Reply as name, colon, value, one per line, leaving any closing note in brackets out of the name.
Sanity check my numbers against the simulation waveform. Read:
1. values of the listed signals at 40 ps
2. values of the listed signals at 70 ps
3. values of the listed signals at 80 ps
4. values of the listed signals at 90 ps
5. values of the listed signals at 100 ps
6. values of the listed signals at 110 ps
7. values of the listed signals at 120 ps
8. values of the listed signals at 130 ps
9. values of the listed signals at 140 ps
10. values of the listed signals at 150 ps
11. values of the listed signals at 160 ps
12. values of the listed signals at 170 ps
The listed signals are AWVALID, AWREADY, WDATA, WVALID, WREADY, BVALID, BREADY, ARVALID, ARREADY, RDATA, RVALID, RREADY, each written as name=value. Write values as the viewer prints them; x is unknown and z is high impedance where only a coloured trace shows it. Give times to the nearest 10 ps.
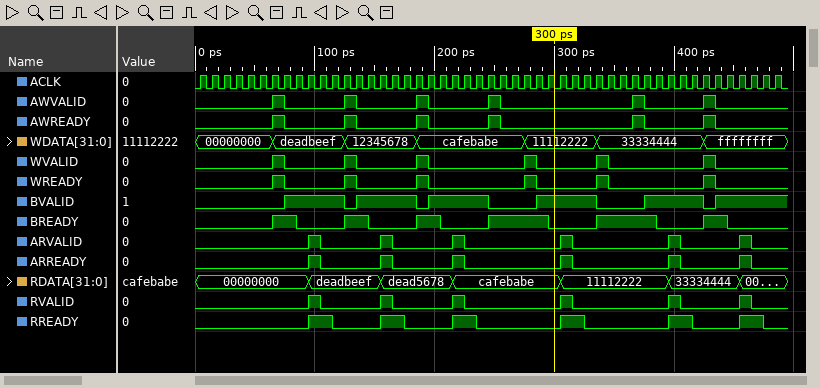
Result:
values of the listed signals at 40 ps: AWVALID=0, AWREADY=0, WDATA=00000000, WVALID=0, WREADY=0, BVALID=0, BREADY=0, ARVALID=0, ARREADY=0, RDATA=00000000, RVALID=0, RREADY=0
values of the listed signals at 70 ps: AWVALID=1, AWREADY=1, WDATA=deadbeef, WVALID=1, WREADY=1, BVALID=0, BREADY=1, ARVALID=0, ARREADY=0, RDATA=00000000, RVALID=0, RREADY=0
values of the listed signals at 80 ps: AWVALID=0, AWREADY=0, WDATA=deadbeef, WVALID=0, WREADY=0, BVALID=1, BREADY=1, ARVALID=0, ARREADY=0, RDATA=00000000, RVALID=0, RREADY=0
values of the listed signals at 90 ps: AWVALID=0, AWREADY=0, WDATA=deadbeef, WVALID=0, WREADY=0, BVALID=1, BREADY=0, ARVALID=0, ARREADY=0, RDATA=00000000, RVALID=0, RREADY=0
values of the listed signals at 100 ps: AWVALID=0, AWREADY=0, WDATA=deadbeef, WVALID=0, WREADY=0, BVALID=1, BREADY=0, ARVALID=1, ARREADY=1, RDATA=deadbeef, RVALID=1, RREADY=1
values of the listed signals at 110 ps: AWVALID=0, AWREADY=0, WDATA=deadbeef, WVALID=0, WREADY=0, BVALID=1, BREADY=0, ARVALID=0, ARREADY=0, RDATA=deadbeef, RVALID=0, RREADY=1
values of the listed signals at 120 ps: AWVALID=0, AWREADY=0, WDATA=deadbeef, WVALID=0, WREADY=0, BVALID=1, BREADY=0, ARVALID=0, ARREADY=0, RDATA=deadbeef, RVALID=0, RREADY=0
values of the listed signals at 130 ps: AWVALID=1, AWREADY=1, WDATA=12345678, WVALID=1, WREADY=1, BVALID=0, BREADY=1, ARVALID=0, ARREADY=0, RDATA=deadbeef, RVALID=0, RREADY=0
values of the listed signals at 140 ps: AWVALID=0, AWREADY=0, WDATA=12345678, WVALID=0, WREADY=0, BVALID=1, BREADY=1, ARVALID=0, ARREADY=0, RDATA=deadbeef, RVALID=0, RREADY=0
values of the listed signals at 150 ps: AWVALID=0, AWREADY=0, WDATA=12345678, WVALID=0, WREADY=0, BVALID=1, BREADY=0, ARVALID=0, ARREADY=0, RDATA=deadbeef, RVALID=0, RREADY=0
values of the listed signals at 160 ps: AWVALID=0, AWREADY=0, WDATA=12345678, WVALID=0, WREADY=0, BVALID=1, BREADY=0, ARVALID=1, ARREADY=1, RDATA=dead5678, RVALID=1, RREADY=1
values of the listed signals at 170 ps: AWVALID=0, AWREADY=0, WDATA=12345678, WVALID=0, WREADY=0, BVALID=1, BREADY=0, ARVALID=0, ARREADY=0, RDATA=dead5678, RVALID=0, RREADY=1
